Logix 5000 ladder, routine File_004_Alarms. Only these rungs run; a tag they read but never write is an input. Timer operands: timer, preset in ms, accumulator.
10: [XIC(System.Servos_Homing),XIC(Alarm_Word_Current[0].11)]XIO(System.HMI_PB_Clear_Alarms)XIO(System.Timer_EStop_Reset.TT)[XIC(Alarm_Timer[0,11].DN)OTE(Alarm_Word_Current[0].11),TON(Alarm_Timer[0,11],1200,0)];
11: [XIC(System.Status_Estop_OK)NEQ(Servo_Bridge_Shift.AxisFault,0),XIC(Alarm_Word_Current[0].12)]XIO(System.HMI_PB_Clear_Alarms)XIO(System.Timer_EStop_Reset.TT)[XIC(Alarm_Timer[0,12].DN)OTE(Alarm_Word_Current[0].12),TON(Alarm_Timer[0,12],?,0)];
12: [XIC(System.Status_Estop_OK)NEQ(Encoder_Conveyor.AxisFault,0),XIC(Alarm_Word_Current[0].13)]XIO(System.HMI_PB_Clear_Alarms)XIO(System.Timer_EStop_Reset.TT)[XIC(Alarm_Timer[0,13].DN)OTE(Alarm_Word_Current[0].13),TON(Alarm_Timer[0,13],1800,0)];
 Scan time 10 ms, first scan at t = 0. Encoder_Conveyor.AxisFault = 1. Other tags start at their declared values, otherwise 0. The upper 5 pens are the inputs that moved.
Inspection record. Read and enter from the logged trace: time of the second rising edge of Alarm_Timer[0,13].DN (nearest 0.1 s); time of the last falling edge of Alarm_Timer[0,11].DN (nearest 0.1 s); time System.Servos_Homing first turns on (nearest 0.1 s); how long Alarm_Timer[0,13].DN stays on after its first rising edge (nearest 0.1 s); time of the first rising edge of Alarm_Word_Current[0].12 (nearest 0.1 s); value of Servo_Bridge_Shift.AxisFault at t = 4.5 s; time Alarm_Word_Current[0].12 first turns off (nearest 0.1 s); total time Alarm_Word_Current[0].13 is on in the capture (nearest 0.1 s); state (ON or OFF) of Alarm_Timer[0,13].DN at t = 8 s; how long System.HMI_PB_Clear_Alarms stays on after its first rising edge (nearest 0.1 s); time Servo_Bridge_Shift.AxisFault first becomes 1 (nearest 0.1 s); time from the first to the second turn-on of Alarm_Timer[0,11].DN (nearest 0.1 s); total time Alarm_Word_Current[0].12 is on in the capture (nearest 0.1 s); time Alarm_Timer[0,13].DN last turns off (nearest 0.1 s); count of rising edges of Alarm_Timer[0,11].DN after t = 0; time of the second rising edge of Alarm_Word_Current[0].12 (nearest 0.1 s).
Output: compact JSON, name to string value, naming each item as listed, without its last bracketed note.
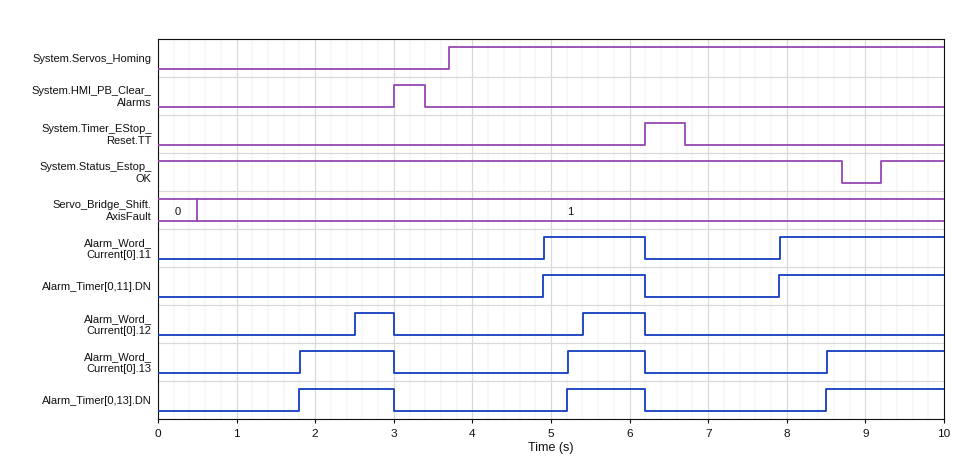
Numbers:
{"time of the second rising edge of Alarm_Timer[0,13].DN": "5.2 s", "time of the last falling edge of Alarm_Timer[0,11].DN": "6.2 s", "time System.Servos_Homing first turns on": "3.7 s", "how long Alarm_Timer[0,13].DN stays on after its first rising edge": "1.2 s", "time of the first rising edge of Alarm_Word_Current[0].12": "2.5 s", "value of Servo_Bridge_Shift.AxisFault at t = 4.5 s": "1", "time Alarm_Word_Current[0].12 first turns off": "3.0 s", "total time Alarm_Word_Current[0].13 is on in the capture": "3.7 s", "state (ON or OFF) of Alarm_Timer[0,13].DN at t = 8 s": "OFF", "how long System.HMI_PB_Clear_Alarms stays on after its first rising edge": "0.4 s", "time Servo_Bridge_Shift.AxisFault first becomes 1": "0.5 s", "time from the first to the second turn-on of Alarm_Timer[0,11].DN": "3.0 s", "total time Alarm_Word_Current[0].12 is on in the capture": "1.3 s", "time Alarm_Timer[0,13].DN last turns off": "6.2 s", "count of rising edges of Alarm_Timer[0,11].DN after t = 0": "2", "time of the second rising edge of Alarm_Word_Current[0].12": "5.4 s"}
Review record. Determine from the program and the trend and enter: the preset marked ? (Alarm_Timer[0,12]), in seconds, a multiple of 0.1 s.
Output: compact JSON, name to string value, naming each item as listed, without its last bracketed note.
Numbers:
{"the preset marked ? (Alarm_Timer[0,12]), in seconds, a multiple of 0.1 s": "2.0 s"}
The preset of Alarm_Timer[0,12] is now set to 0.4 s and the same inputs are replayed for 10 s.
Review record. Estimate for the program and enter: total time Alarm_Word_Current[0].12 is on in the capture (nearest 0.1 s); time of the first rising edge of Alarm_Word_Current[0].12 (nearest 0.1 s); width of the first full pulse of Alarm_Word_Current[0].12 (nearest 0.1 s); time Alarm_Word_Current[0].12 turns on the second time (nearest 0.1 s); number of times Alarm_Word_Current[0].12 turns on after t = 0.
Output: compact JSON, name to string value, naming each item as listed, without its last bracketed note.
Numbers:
{"total time Alarm_Word_Current[0].12 is on in the capture": "7.4 s", "time of the first rising edge of Alarm_Word_Current[0].12": "0.9 s", "width of the first full pulse of Alarm_Word_Current[0].12": "2.1 s", "time Alarm_Word_Current[0].12 turns on the second time": "3.8 s", "number of times Alarm_Word_Current[0].12 turns on after t = 0": "3"}
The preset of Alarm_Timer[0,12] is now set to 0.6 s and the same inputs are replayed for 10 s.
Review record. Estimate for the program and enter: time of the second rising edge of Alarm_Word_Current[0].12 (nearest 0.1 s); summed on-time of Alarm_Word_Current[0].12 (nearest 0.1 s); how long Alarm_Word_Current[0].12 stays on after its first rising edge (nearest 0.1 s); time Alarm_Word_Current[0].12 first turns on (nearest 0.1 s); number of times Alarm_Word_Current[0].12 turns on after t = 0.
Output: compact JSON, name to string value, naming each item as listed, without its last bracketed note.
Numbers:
{"time of the second rising edge of Alarm_Word_Current[0].12": "4.0 s", "summed on-time of Alarm_Word_Current[0].12": "6.8 s", "how long Alarm_Word_Current[0].12 stays on after its first rising edge": "1.9 s", "time Alarm_Word_Current[0].12 first turns on": "1.1 s", "number of times Alarm_Word_Current[0].12 turns on after t = 0": "3"}
